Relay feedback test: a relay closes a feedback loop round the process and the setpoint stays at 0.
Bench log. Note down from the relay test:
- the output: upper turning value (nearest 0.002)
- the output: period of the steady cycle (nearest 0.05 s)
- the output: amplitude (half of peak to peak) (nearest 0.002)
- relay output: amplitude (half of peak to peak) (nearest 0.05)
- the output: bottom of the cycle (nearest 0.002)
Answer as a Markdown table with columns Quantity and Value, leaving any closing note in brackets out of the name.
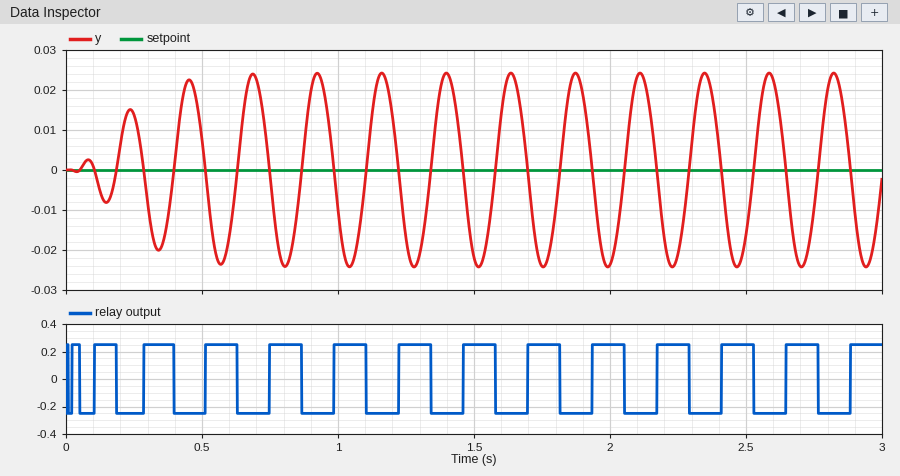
| Quantity | Value |
|---|---|
| the output: upper turning value | 0.024 |
| the output: period of the steady cycle | 0.25 s |
| the output: amplitude (half of peak to peak) | 0.024 |
| relay output: amplitude (half of peak to peak) | 0.25 |
| the output: bottom of the cycle | -0.024 |
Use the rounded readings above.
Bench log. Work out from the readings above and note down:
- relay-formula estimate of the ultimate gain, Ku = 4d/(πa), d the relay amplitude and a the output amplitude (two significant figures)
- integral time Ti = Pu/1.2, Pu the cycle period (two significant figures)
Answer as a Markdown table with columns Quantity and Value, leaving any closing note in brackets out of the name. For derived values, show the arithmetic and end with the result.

| Quantity | Value |
|---|---|
| relay-formula estimate of the ultimate gain, Ku = 4d/(πa), d the relay amplitude and a the output amplitude | 4 × 0.25 / (π × 0.024) = 13 |
| integral time Ti = Pu/1.2, Pu the cycle period | 0.25 / 1.2 = 0.21 s |
